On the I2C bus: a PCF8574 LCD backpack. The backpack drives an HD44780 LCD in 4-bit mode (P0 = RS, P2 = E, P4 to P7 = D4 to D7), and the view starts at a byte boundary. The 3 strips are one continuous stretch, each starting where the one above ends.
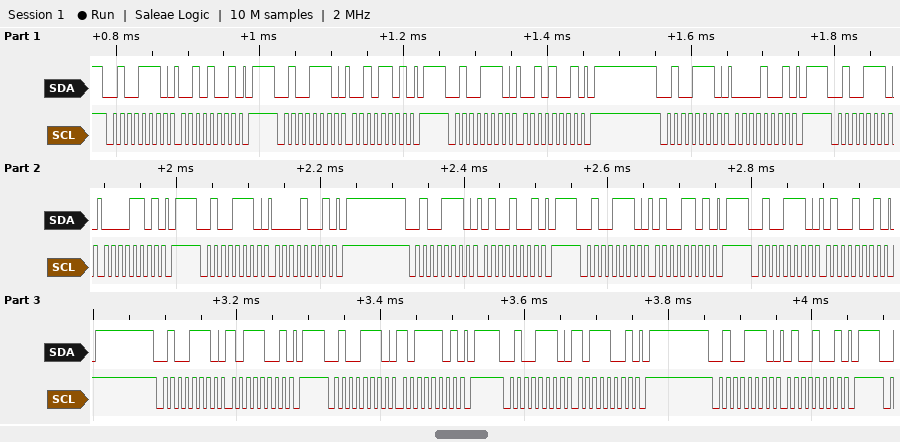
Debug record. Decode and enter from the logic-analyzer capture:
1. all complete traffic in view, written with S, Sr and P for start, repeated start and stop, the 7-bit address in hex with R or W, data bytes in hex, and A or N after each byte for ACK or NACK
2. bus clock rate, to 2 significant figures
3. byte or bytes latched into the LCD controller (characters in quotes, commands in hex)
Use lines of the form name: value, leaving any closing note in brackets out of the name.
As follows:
all complete traffic in view, written with S, Sr and P for start, repeated start and stop, the 7-bit address in hex with R or W, data bytes in hex, and A or N after each byte for ACK or NACK: S 27W A 29 A P S 27W A 2D A P S 27W A 29 A P S 27W A 09 A P S 27W A 0D A P S 27W A 09 A P S 27W A 49 A P S 27W A 4D A P S 27W A 49 A P S 27W A B9 A P S 27W A BD A P S 27W A B9 A P S 27W A 49 A P
bus clock rate, to 2 significant figures: 100 kHz
byte or bytes latched into the LCD controller: ' ' 'K'
